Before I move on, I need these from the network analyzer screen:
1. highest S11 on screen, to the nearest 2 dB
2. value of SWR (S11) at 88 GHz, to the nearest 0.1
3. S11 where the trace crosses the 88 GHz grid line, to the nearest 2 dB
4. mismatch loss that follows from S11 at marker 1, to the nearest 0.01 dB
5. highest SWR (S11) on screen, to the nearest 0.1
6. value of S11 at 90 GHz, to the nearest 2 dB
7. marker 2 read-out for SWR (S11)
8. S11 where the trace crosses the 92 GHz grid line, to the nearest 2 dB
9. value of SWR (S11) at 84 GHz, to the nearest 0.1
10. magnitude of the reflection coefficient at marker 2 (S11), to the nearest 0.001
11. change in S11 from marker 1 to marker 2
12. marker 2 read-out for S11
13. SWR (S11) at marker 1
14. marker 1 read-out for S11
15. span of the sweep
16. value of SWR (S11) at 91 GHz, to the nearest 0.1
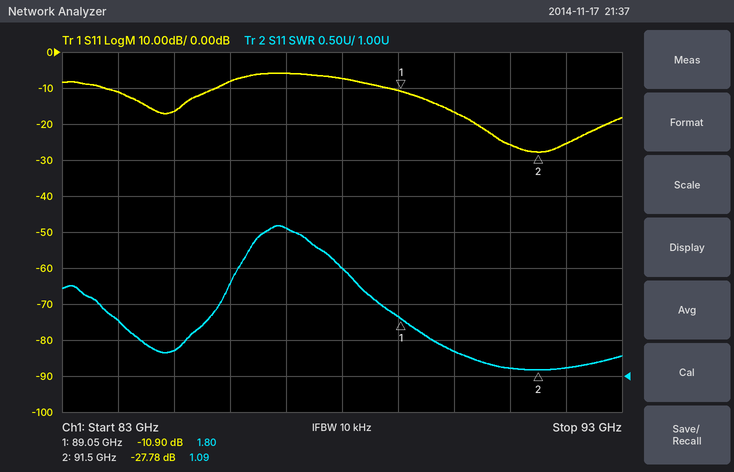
-6 dB
2.5
-8 dB
0.37 dB
3.1
-16 dB
1.09
-26 dB
1.8
0.041
-16.88 dB
-27.78 dB
1.80
-10.90 dB
10 GHz
1.1
